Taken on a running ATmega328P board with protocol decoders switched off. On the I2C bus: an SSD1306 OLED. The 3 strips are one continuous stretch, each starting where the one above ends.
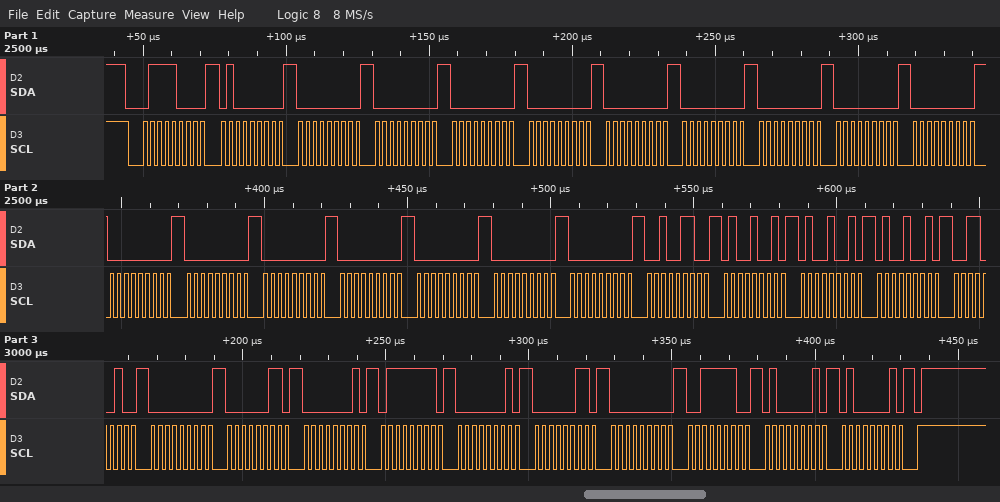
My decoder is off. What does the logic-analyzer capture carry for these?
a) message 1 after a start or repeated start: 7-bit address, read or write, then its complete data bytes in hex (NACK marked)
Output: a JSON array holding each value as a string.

["0x3C write: 40 00 00 00 00 00 00 00 00 00 00 00 00 00 00 00 00 26 49 49 49 32 00 03 01 7F 01 03 00 3E 41 41"]
